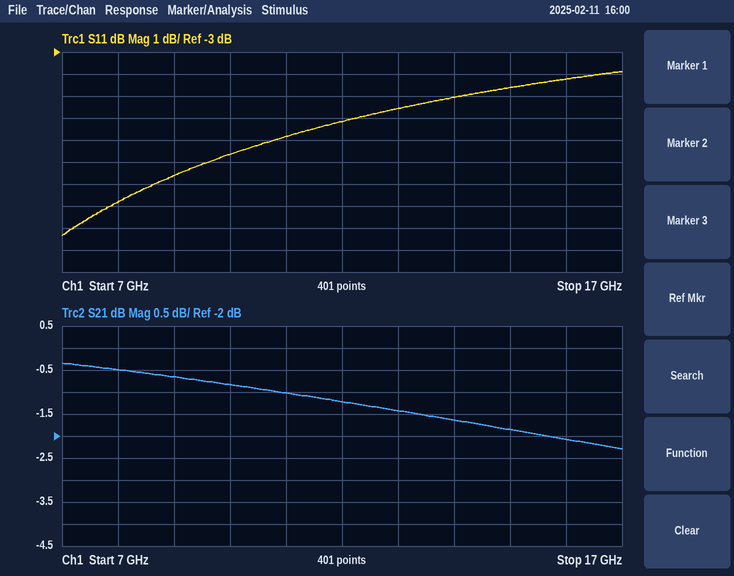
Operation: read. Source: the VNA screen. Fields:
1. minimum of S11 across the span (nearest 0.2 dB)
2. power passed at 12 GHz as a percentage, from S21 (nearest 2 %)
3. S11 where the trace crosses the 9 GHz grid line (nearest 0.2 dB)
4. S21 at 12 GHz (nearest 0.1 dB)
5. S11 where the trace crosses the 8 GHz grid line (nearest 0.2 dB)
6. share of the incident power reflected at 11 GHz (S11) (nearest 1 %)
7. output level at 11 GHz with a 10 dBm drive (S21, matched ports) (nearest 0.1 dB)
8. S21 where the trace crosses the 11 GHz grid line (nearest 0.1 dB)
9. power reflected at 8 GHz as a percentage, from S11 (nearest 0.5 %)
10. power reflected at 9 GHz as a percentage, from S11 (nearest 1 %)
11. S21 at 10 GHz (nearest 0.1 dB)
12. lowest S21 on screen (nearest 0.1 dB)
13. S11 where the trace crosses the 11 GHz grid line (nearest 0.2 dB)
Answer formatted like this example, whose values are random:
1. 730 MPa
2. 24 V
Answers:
1. -11.4 dB
2. 76 %
3. -8.6 dB
4. -1.2 dB
5. -9.8 dB
6. 21 %
7. 9.0 dBm
8. -1.0 dB
9. 10.5 %
10. 14 %
11. -0.8 dB
12. -2.3 dB
13. -6.8 dB
